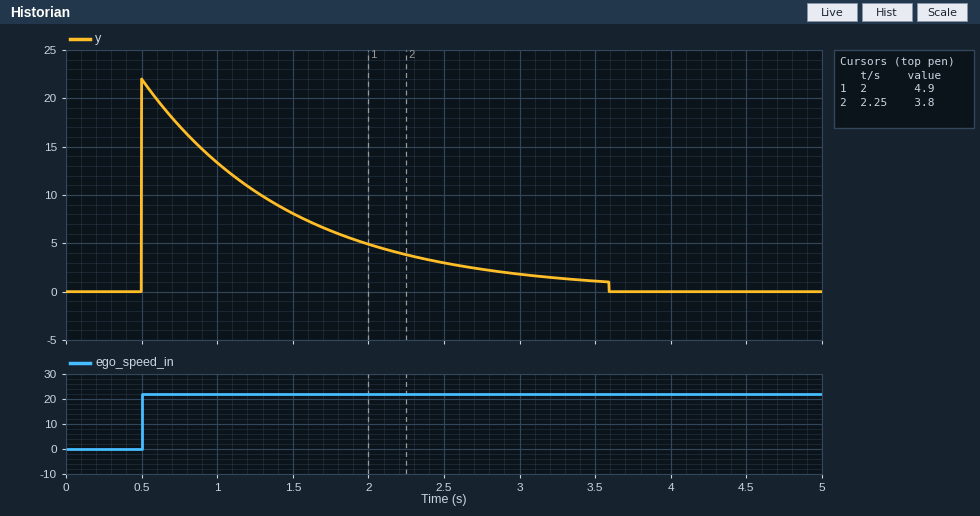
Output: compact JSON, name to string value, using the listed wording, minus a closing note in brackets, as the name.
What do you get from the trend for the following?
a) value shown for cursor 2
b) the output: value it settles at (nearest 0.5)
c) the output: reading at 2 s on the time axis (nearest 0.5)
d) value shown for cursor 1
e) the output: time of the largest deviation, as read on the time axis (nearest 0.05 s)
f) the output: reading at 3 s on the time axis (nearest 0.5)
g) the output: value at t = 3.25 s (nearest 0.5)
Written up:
{"value shown for cursor 2": "3.8", "the output: value it settles at": "0.0", "the output: reading at 2 s on the time axis": "5.0", "value shown for cursor 1": "4.9", "the output: time of the largest deviation, as read on the time axis": "0.50 s", "the output: reading at 3 s on the time axis": "2.0", "the output: value at t = 3.25 s": "1.5"}
